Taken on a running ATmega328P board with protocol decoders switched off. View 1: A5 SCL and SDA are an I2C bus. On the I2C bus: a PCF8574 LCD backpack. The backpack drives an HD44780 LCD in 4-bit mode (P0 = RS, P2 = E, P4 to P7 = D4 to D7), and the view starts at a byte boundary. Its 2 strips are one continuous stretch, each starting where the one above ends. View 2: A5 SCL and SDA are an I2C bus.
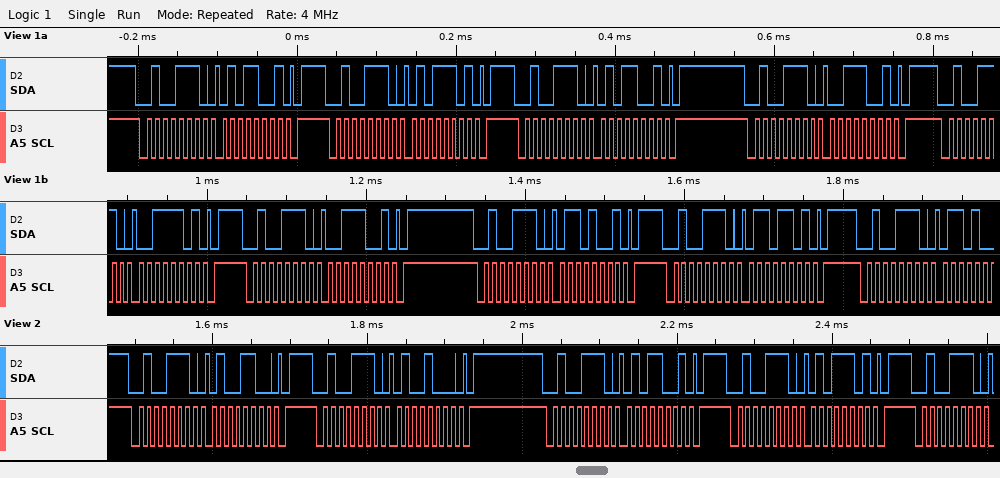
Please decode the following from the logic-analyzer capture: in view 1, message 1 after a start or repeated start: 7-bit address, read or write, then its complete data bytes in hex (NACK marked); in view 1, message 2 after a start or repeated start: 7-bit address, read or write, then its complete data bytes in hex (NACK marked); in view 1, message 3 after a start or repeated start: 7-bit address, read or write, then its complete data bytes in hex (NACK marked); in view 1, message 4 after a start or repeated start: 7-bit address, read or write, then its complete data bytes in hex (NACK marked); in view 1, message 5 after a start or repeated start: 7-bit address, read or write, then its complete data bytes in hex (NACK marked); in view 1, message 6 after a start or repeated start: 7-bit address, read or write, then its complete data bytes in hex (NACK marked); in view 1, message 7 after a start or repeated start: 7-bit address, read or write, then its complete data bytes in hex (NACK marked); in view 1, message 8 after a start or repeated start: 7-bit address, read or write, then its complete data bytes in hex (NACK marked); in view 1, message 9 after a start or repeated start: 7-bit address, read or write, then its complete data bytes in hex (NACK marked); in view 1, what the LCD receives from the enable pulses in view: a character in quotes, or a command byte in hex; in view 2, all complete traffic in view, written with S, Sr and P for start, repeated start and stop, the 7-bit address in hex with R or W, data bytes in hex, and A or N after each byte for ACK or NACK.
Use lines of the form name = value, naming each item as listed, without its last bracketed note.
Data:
in view 1, message 1 after a start or repeated start: 7-bit address, read or write, then its complete data bytes in hex = 0x27 write: 59
in view 1, message 2 after a start or repeated start: 7-bit address, read or write, then its complete data bytes in hex = 0x27 write: 5D
in view 1, message 3 after a start or repeated start: 7-bit address, read or write, then its complete data bytes in hex = 0x27 write: 59
in view 1, message 4 after a start or repeated start: 7-bit address, read or write, then its complete data bytes in hex = 0x27 write: 39
in view 1, message 5 after a start or repeated start: 7-bit address, read or write, then its complete data bytes in hex = 0x27 write: 3D
in view 1, message 6 after a start or repeated start: 7-bit address, read or write, then its complete data bytes in hex = 0x27 write: 39
in view 1, message 7 after a start or repeated start: 7-bit address, read or write, then its complete data bytes in hex = 0x27 write: 69
in view 1, message 8 after a start or repeated start: 7-bit address, read or write, then its complete data bytes in hex = 0x27 write: 6D
in view 1, message 9 after a start or repeated start: 7-bit address, read or write, then its complete data bytes in hex = 0x27 write
in view 1, what the LCD receives from the enable pulses in view: a character in quotes, or a command byte in hex = 'S'
in view 2, all complete traffic in view, written with S, Sr and P for start, repeated start and stop, the 7-bit address in hex with R or W, data bytes in hex, and A or N after each byte for ACK or NACK = S 27W A 4C A P S 27W A 48 A P S 27W A 59 A P S 27W A 5D A P S 27W A
